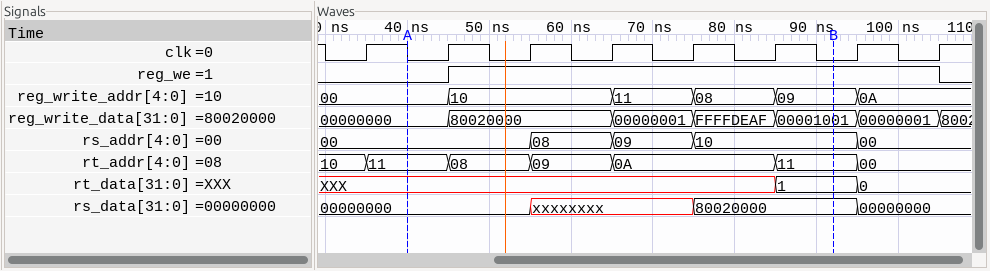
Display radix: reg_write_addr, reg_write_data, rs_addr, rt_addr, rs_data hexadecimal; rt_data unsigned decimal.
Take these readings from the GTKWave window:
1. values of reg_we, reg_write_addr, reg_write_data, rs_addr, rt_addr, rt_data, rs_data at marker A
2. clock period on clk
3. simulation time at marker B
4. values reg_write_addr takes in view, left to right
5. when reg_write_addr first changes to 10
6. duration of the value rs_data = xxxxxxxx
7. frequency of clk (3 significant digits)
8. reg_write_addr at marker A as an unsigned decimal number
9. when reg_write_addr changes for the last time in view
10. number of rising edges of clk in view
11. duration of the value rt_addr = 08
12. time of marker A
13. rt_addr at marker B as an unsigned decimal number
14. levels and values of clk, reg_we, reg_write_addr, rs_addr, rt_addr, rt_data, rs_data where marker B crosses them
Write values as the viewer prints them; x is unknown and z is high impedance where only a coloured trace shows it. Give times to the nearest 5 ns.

reg_we=0, reg_write_addr=00, reg_write_data=00000000, rs_addr=00, rt_addr=11, rt_data=XXX, rs_data=00000000
10 ns
90 ns
00, 10, 11, 08, 09, 0A
45 ns
20 ns
100 MHz
0
95 ns
8
10 ns
40 ns
17
clk=0, reg_we=1, reg_write_addr=09, rs_addr=10, rt_addr=11, rt_data=1, rs_data=80020000
